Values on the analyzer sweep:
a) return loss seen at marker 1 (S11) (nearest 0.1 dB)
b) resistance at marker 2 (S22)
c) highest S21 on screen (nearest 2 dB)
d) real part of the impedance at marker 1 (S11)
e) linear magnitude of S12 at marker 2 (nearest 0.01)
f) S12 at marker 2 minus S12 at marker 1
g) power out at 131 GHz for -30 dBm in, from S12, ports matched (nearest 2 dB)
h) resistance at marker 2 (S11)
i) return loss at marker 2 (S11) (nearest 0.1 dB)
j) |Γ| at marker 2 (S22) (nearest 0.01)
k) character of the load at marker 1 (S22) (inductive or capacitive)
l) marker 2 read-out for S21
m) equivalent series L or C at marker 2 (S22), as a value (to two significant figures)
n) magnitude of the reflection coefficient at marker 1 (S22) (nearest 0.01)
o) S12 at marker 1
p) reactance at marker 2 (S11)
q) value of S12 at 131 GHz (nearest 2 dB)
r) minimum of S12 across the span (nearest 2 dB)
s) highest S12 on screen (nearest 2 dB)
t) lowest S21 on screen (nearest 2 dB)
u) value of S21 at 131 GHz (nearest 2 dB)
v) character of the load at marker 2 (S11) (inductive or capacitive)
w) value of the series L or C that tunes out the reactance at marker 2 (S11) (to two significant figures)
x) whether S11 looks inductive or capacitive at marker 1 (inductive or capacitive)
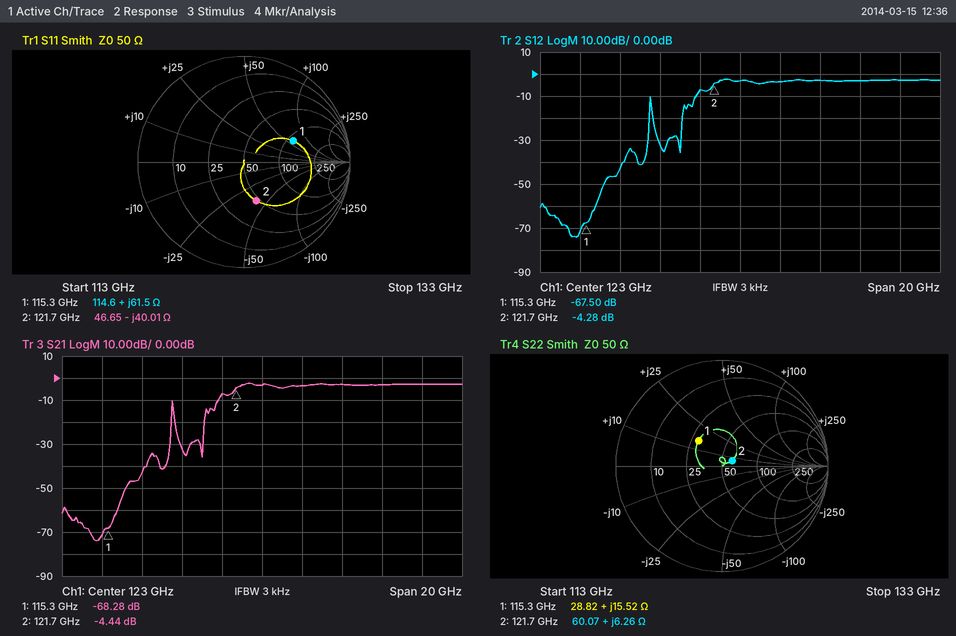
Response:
5.9 dB
60.07 Ω
-2 dB
114.6 Ω
0.61
63.22 dB
-32 dBm
46.65 Ω
8.3 dB
0.11
inductive
-4.44 dB
8.2 pH
0.33
-67.50 dB
-40.01 Ω
-2 dB
-74 dB
-2 dB
-74 dB
-2 dB
capacitive
52 pH
inductive
